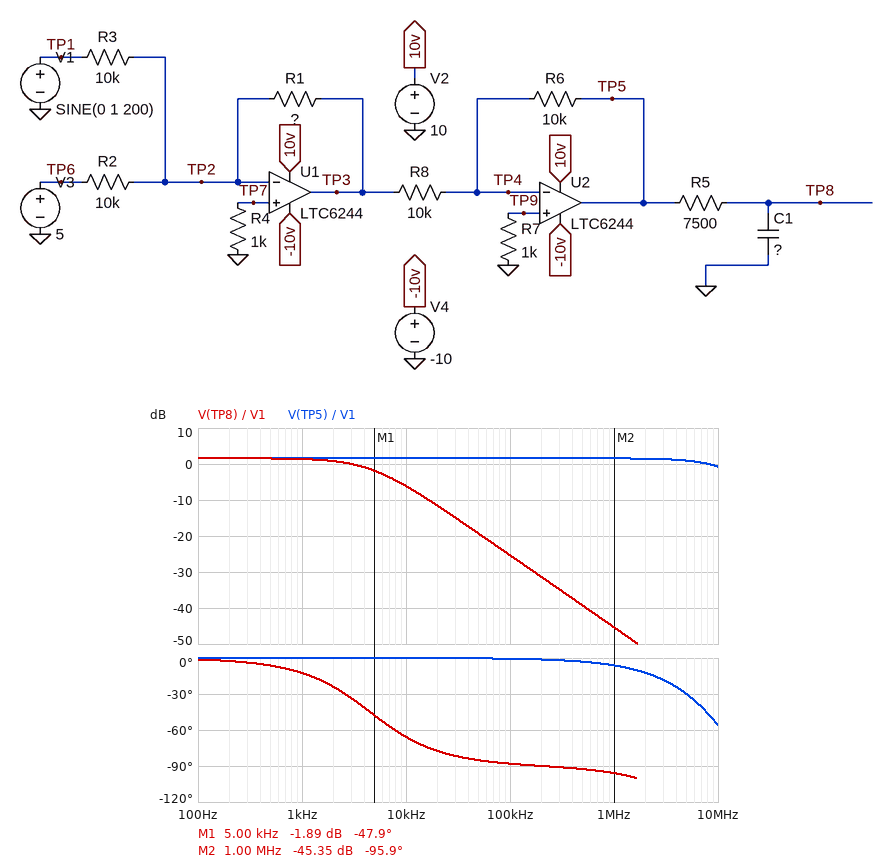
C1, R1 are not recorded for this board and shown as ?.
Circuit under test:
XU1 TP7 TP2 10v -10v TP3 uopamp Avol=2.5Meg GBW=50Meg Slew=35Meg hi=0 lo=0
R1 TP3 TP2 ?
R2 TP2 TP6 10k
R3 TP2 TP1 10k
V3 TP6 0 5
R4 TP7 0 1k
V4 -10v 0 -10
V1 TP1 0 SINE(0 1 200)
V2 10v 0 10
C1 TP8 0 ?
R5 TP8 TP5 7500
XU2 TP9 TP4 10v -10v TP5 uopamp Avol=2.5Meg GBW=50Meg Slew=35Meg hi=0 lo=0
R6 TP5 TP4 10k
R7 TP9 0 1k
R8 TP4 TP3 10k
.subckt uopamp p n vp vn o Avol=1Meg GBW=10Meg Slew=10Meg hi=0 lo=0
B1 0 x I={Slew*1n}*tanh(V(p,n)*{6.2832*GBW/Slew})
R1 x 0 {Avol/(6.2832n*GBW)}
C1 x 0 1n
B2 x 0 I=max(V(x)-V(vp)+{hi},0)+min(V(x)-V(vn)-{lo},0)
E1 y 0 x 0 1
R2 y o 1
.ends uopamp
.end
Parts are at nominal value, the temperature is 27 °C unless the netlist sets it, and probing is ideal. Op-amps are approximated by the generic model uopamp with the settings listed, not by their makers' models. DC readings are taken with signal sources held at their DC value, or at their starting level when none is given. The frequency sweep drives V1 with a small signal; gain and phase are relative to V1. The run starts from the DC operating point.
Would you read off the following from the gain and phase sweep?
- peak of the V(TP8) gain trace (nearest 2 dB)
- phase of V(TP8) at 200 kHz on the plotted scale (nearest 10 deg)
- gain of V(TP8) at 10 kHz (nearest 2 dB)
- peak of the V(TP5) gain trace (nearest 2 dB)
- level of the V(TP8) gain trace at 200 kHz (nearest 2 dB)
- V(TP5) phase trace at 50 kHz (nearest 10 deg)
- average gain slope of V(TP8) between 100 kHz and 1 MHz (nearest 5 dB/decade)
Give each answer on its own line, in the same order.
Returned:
2 dB
-90 deg
-6 dB
2 dB
-32 dB
0 deg
-20 dB/decade
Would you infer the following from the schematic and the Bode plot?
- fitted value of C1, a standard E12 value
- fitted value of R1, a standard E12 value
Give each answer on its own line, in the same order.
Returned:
4.7 nF
12 kΩ
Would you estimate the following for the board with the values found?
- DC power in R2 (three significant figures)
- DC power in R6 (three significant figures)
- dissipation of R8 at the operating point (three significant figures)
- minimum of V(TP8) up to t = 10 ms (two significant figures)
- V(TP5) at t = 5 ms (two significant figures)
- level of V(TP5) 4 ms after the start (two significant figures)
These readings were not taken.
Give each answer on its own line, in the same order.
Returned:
2.50 mW
3.60 mW
3.60 mW
4.8 V
6.0 V
4.9 V
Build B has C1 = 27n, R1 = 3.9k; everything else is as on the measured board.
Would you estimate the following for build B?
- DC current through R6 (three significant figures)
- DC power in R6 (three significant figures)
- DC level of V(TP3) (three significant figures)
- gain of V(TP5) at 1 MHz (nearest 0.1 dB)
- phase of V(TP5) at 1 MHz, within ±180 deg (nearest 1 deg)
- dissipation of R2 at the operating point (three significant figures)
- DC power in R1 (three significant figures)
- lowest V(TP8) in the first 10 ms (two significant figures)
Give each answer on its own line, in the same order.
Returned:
195 µA
380 µW
-1.95 V
-8.2 dB
-4 deg
2.50 mW
975 µW
1.6 V
